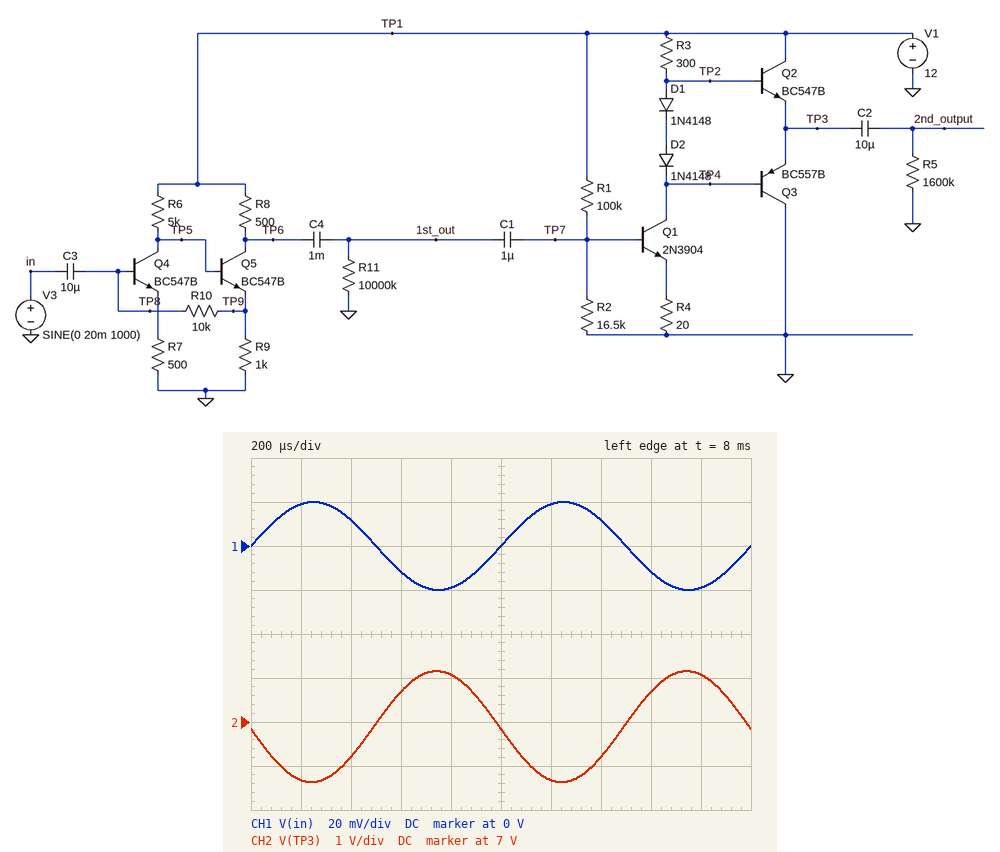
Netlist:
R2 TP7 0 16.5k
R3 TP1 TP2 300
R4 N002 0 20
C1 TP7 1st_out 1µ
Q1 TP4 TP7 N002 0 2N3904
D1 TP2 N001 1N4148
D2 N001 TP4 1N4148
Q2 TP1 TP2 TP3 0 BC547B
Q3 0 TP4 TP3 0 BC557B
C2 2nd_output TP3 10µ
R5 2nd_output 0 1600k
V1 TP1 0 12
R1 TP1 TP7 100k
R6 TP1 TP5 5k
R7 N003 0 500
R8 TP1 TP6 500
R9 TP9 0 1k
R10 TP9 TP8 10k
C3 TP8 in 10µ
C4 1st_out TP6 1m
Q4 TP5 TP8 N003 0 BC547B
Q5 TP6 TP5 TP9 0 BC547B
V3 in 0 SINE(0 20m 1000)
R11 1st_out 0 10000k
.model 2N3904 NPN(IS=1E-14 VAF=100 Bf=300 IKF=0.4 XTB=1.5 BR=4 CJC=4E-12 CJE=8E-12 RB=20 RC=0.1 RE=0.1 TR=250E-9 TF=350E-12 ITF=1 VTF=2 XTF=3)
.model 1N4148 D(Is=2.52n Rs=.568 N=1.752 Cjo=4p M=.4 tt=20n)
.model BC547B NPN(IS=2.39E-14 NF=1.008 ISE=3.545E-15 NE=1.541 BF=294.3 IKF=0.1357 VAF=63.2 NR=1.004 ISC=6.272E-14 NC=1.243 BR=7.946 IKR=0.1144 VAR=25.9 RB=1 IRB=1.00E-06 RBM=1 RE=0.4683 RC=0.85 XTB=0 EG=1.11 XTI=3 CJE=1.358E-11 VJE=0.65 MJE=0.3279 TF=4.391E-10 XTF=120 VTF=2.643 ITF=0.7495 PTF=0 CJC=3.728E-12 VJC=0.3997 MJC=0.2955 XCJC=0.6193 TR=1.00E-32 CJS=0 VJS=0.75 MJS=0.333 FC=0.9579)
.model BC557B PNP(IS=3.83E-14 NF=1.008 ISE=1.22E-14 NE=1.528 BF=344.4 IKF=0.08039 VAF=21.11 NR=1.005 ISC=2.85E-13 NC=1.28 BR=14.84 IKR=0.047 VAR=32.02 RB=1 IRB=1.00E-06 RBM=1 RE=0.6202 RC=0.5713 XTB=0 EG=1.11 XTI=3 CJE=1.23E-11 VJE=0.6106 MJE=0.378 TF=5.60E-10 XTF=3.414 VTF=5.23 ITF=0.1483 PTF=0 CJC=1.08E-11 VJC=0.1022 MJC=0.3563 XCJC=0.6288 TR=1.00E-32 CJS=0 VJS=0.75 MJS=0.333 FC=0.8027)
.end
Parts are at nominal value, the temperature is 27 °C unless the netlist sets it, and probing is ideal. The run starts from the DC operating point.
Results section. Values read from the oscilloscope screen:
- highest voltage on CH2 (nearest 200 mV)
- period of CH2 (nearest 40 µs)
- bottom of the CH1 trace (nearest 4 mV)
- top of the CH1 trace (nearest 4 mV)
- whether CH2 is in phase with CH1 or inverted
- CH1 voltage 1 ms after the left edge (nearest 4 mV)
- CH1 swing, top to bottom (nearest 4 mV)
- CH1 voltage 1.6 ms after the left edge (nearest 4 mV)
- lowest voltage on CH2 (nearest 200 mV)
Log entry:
8.2 V
1.00 ms
-20 mV
20 mV
inverted
0 V
40 mV
-12 mV
5.6 V
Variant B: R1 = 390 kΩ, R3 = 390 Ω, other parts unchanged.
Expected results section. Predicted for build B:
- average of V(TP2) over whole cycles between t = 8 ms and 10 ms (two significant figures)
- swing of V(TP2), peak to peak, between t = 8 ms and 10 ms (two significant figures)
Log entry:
12 V
28 mV
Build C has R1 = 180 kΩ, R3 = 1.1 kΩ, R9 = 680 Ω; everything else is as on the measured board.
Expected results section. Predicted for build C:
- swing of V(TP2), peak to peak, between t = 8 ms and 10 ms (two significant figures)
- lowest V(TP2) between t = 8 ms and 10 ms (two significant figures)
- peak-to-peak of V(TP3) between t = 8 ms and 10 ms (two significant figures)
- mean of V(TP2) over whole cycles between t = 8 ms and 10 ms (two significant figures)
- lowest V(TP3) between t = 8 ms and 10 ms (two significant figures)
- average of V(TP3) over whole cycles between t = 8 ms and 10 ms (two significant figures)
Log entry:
9.8 V
1.7 V
9.9 V
7.0 V
1.0 V
6.3 V
